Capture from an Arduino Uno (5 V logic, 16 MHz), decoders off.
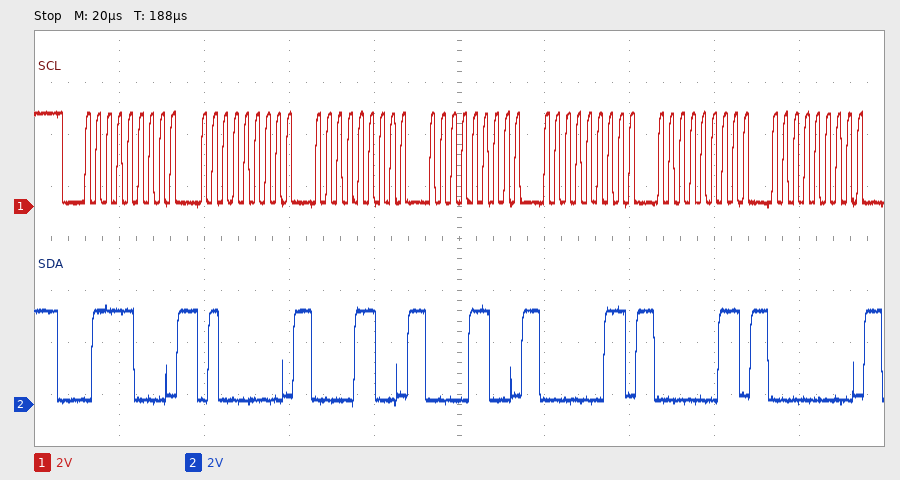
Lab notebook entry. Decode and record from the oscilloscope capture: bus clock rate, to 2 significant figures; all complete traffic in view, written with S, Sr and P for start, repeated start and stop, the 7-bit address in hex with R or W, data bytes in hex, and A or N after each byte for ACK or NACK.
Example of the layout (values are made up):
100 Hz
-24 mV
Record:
400 kHz
S 3CW A 40 A 0C A 0C A 03 A 03 A 00 A
